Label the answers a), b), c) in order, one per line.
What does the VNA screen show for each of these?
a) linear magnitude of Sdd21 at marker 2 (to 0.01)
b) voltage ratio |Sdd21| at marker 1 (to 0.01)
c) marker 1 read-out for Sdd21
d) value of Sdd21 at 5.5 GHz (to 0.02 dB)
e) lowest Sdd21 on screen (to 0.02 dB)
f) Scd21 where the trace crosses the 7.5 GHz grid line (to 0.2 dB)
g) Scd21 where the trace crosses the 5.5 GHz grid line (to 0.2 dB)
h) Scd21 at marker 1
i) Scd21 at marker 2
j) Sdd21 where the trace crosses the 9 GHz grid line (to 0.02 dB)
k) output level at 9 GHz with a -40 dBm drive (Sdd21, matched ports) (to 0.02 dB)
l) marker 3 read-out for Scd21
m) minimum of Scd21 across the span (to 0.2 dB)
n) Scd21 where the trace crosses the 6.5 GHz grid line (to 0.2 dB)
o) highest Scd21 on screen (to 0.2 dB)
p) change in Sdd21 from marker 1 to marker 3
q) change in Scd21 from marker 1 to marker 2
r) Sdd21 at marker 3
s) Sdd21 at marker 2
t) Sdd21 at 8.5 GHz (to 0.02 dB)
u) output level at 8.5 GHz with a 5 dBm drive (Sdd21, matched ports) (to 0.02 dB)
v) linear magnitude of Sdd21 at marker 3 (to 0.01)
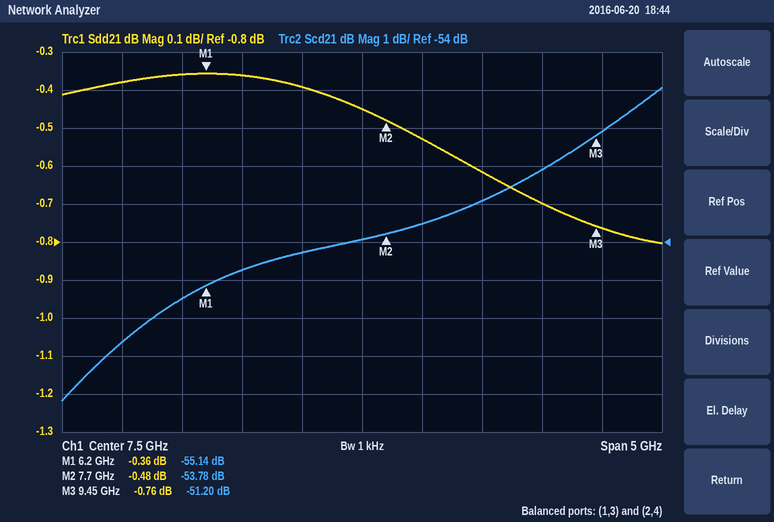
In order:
a) 0.95
b) 0.96
c) -0.36 dB
d) -0.38 dB
e) -0.80 dB
f) -54.0 dB
g) -56.6 dB
h) -55.14 dB
i) -53.78 dB
j) -0.70 dB
k) -40.70 dBm
l) -51.20 dB
m) -58.2 dB
n) -54.8 dB
o) -50.0 dB
p) -0.40 dB
q) 1.36 dB
r) -0.76 dB
s) -0.48 dB
t) -0.62 dB
u) 4.38 dBm
v) 0.92
